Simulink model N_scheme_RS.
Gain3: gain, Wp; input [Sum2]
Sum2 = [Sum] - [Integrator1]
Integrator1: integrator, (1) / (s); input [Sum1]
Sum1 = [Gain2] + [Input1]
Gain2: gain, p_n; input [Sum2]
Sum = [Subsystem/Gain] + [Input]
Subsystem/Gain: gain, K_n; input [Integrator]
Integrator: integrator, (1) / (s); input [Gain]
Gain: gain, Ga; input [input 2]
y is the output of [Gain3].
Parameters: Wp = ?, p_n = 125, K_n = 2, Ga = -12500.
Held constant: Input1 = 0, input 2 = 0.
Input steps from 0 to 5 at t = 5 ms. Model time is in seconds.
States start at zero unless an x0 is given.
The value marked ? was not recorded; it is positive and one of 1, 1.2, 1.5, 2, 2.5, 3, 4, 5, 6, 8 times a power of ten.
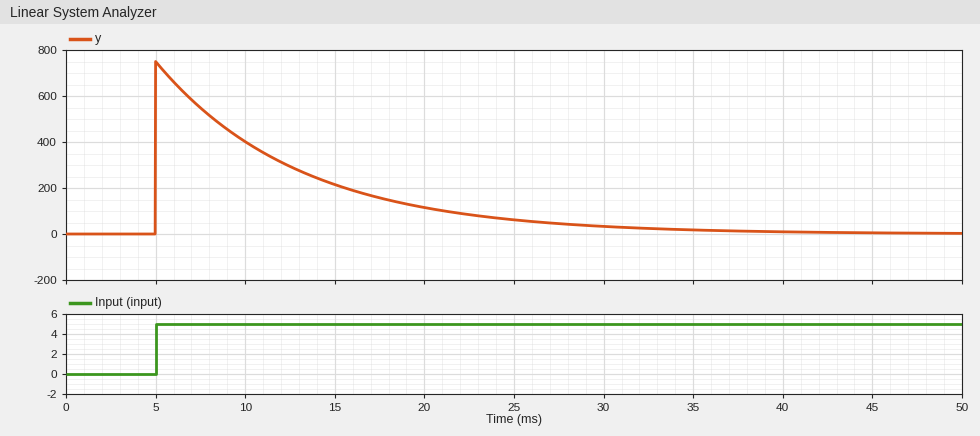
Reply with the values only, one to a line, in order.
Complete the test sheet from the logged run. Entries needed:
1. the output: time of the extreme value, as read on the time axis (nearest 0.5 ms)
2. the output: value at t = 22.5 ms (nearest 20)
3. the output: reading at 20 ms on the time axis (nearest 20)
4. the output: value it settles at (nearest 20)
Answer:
5.0 ms
80
120
0
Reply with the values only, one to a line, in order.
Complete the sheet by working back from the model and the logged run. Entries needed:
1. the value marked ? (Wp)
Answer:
150
